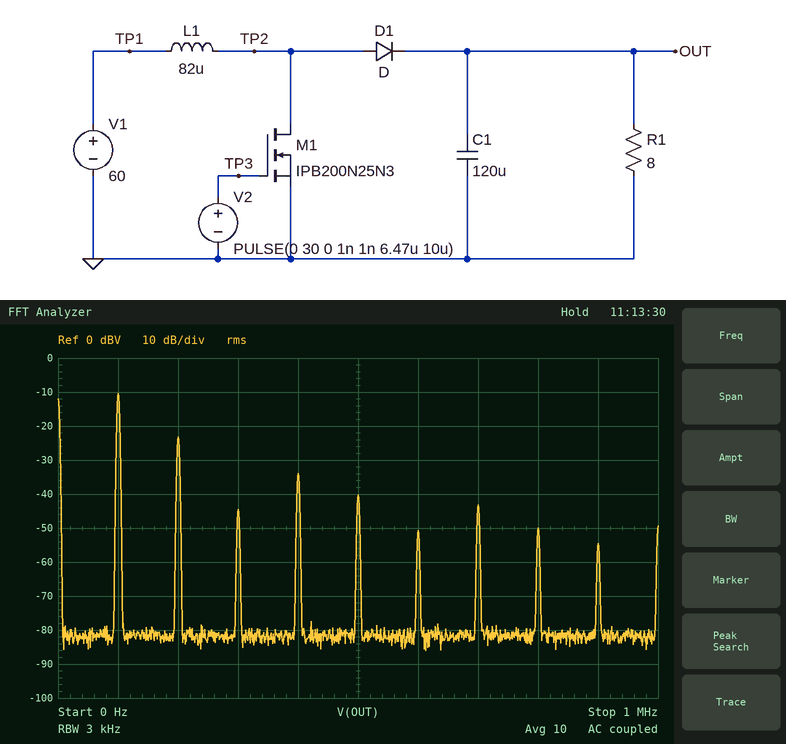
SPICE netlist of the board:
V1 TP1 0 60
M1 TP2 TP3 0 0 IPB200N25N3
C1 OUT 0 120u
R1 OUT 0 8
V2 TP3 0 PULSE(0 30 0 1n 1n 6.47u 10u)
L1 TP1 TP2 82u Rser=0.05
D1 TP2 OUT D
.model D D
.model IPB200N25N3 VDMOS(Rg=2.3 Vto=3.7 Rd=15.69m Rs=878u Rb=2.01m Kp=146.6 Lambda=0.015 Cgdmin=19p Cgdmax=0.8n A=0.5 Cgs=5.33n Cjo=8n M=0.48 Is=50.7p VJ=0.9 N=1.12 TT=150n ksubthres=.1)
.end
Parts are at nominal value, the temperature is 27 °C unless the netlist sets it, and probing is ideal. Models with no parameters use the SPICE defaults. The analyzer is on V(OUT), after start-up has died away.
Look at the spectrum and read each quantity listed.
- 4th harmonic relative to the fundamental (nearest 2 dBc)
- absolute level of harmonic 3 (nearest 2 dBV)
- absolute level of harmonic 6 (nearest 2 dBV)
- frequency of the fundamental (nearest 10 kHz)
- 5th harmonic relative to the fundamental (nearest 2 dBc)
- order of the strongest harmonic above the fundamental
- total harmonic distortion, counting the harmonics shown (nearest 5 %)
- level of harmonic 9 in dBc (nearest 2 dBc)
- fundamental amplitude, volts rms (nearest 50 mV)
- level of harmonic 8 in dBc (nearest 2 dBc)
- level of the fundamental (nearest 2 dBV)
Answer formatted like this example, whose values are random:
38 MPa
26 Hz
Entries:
-24 dBc
-44 dBV
-50 dBV
100 kHz
-30 dBc
2
25 %
-44 dBc
300 mV
-40 dBc
-10 dBV
